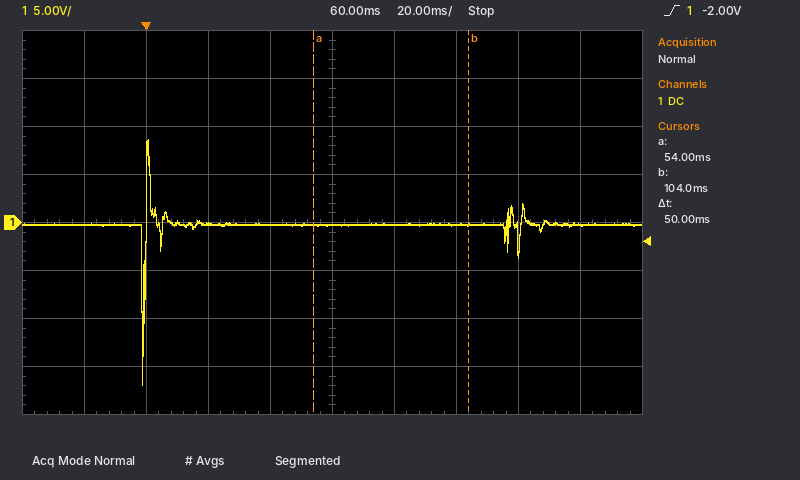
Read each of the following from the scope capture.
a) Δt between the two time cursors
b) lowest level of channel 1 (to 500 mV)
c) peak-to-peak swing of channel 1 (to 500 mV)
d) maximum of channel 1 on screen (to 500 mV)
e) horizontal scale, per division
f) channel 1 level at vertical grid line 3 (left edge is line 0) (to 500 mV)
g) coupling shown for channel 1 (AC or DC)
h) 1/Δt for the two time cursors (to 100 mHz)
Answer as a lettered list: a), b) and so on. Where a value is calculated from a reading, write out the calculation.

a) 50 ms
b) -17.0 V
c) 8.5 V − (-17.0 V) = 25.5 V
d) 8.5 V
e) 20 ms
f) 0.0 V
g) DC
h) 1 / 50 ms ≈ 20.0 Hz
